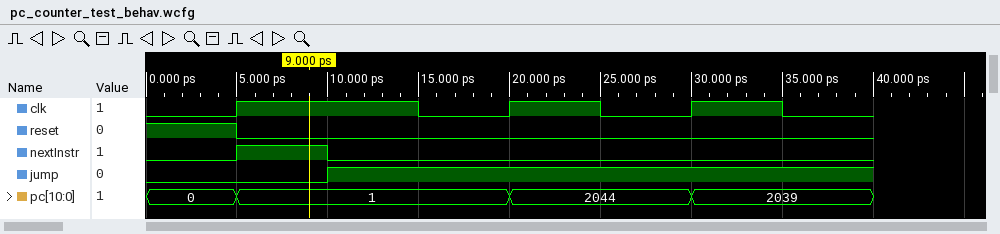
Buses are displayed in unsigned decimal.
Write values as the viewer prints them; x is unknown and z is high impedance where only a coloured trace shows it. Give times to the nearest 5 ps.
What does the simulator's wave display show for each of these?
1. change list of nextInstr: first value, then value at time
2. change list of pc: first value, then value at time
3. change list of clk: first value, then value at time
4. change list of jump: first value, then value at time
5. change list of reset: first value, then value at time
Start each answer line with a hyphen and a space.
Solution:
- 0, 1 at 5 ps, 0 at 10 ps
- 0, 1 at 5 ps, 2044 at 20 ps, 2039 at 30 ps
- 0, 1 at 5 ps, 0 at 15 ps, 1 at 20 ps, 0 at 25 ps, 1 at 30 ps, 0 at 35 ps
- 0, 1 at 10 ps
- 1, 0 at 5 ps
